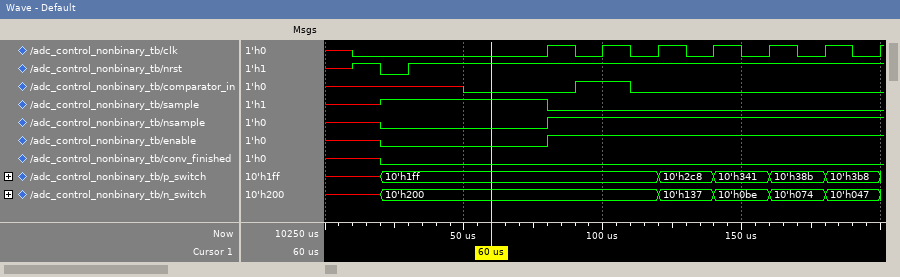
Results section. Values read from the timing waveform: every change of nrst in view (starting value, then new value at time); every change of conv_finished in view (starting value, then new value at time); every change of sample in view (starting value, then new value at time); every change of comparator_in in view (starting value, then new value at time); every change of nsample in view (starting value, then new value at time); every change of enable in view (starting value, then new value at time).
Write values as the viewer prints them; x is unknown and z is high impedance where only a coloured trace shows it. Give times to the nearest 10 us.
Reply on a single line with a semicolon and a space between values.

x, 1 at 10 us, 0 at 20 us, 1 at 30 us; x, 0 at 20 us; x, 1 at 20 us, 0 at 80 us; x, 0 at 50 us, 1 at 90 us, 0 at 110 us; x, 0 at 20 us, 1 at 80 us; x, 0 at 20 us, 1 at 80 us
